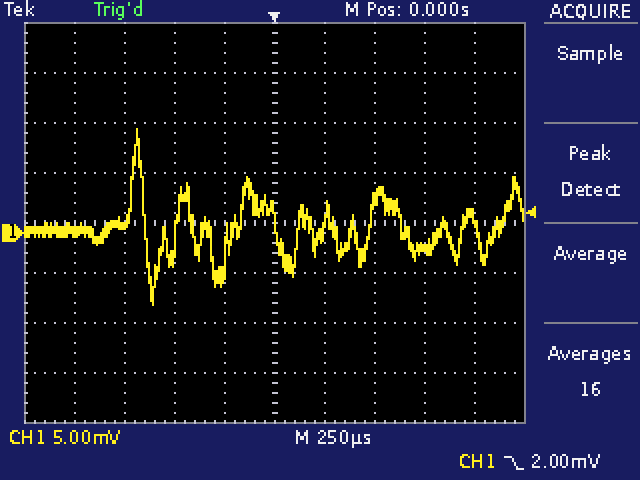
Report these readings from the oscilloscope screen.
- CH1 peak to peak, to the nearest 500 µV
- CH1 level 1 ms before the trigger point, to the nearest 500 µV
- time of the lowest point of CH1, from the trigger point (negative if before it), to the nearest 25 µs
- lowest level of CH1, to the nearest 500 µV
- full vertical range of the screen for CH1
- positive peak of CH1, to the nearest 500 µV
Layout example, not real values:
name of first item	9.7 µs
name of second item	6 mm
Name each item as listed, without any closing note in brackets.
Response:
CH1 peak to peak, to the nearest 500 µV	17.5 mV
CH1 level 1 ms before the trigger point, to the nearest 500 µV	0.0 mV
time of the lowest point of CH1, from the trigger point (negative if before it), to the nearest 25 µs	-600 µs
lowest level of CH1, to the nearest 500 µV	-7.0 mV
full vertical range of the screen for CH1	40 mV
positive peak of CH1, to the nearest 500 µV	10.5 mV
